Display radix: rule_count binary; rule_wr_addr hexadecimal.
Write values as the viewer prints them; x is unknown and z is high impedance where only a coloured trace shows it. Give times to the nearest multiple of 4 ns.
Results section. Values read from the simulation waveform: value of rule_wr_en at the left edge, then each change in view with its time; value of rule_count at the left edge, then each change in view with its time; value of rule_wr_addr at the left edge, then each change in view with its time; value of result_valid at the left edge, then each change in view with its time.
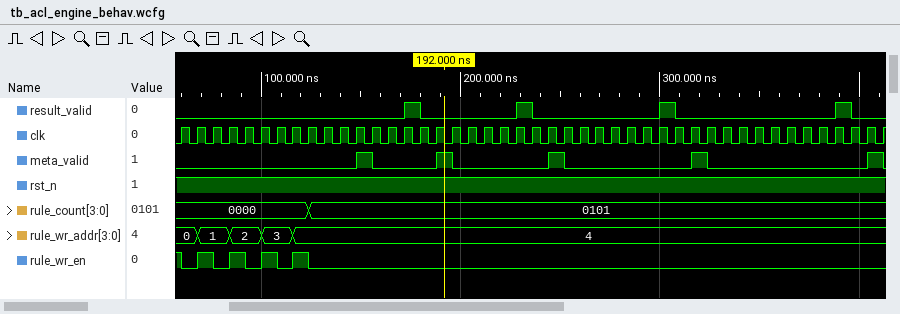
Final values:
1, 0 at 60 ns, 1 at 68 ns, 0 at 76 ns, 1 at 84 ns, 0 at 92 ns, 1 at 100 ns, 0 at 108 ns, 1 at 116 ns, 0 at 124 ns
0000, 0101 at 124 ns
0, 1 at 68 ns, 2 at 84 ns, 3 at 100 ns, 4 at 116 ns
0, 1 at 172 ns, 0 at 180 ns, 1 at 228 ns, 0 at 236 ns, 1 at 300 ns, 0 at 308 ns, 1 at 388 ns, 0 at 396 ns
